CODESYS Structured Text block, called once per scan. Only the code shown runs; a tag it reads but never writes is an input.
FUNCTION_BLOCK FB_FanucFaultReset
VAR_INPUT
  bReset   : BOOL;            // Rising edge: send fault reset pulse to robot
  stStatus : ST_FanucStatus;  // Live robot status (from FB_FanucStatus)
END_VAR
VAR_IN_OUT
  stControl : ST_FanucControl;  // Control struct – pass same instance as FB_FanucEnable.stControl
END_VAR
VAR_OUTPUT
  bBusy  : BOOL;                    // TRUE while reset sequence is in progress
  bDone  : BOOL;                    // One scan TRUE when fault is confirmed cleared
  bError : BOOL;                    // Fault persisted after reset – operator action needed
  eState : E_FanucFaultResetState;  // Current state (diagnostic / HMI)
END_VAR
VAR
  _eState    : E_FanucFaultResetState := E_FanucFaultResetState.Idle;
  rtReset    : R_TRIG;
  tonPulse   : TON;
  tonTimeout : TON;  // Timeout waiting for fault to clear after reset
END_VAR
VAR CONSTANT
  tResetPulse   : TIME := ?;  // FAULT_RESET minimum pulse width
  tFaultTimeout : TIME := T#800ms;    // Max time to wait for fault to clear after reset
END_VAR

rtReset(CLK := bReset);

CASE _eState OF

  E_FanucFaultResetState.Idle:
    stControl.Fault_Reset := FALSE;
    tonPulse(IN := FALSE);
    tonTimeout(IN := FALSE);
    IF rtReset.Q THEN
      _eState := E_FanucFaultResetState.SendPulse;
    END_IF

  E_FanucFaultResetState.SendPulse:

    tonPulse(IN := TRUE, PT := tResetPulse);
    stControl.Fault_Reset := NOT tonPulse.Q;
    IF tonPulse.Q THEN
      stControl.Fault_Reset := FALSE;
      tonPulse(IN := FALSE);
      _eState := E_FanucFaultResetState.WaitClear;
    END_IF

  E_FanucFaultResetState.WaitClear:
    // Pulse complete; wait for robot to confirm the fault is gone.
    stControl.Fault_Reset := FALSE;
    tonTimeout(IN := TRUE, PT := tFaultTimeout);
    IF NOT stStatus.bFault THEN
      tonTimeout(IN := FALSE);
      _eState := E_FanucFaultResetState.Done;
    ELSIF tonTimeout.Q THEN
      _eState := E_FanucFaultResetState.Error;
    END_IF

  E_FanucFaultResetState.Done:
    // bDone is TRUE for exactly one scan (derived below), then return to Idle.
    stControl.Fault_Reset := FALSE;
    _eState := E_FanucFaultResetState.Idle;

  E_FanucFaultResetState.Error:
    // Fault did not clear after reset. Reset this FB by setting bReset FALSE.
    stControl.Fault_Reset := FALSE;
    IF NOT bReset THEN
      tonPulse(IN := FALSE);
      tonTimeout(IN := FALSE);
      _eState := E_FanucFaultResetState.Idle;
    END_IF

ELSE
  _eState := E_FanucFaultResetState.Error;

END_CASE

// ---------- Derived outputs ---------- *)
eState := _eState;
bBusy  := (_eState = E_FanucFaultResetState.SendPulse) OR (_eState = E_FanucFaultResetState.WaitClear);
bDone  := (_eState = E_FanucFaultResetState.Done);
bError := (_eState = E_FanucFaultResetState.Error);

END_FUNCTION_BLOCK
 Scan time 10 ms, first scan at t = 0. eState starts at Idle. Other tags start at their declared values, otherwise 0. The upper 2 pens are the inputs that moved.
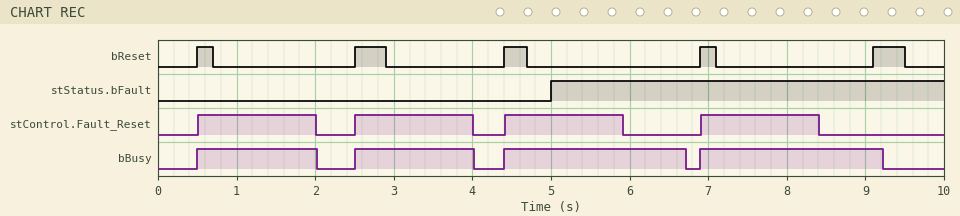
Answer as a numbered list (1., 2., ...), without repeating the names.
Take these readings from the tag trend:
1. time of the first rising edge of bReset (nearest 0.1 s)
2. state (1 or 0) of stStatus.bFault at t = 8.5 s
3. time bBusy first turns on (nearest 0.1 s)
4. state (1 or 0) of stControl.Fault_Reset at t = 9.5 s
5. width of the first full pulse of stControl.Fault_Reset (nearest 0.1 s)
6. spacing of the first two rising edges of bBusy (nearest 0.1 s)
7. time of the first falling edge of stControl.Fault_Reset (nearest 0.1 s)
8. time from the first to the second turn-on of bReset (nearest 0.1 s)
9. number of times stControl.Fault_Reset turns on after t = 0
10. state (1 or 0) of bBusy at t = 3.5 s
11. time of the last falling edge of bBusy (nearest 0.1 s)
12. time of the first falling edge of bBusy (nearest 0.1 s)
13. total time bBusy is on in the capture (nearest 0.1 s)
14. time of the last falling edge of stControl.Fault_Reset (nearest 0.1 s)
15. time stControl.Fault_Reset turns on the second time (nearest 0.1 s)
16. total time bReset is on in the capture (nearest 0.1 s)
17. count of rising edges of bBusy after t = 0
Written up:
1. 0.5 s
2. 1
3. 0.5 s
4. 0
5. 1.5 s
6. 2.0 s
7. 2.0 s
8. 2.0 s
9. 4
10. 1
11. 9.2 s
12. 2.0 s
13. 7.7 s
14. 8.4 s
15. 2.5 s
16. 1.5 s
17. 4
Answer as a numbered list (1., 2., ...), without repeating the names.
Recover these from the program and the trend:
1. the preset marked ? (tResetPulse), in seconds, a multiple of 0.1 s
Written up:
1. 1.5 s
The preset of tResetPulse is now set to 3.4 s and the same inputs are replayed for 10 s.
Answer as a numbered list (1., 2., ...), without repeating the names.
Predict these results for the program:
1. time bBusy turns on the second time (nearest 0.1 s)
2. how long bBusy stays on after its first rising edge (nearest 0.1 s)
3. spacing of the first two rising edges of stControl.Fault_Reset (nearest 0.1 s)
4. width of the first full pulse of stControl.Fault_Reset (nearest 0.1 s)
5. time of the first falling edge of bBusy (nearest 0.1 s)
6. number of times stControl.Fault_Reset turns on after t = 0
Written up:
1. 4.4 s
2. 3.4 s
3. 3.9 s
4. 3.4 s
5. 3.9 s
6. 3
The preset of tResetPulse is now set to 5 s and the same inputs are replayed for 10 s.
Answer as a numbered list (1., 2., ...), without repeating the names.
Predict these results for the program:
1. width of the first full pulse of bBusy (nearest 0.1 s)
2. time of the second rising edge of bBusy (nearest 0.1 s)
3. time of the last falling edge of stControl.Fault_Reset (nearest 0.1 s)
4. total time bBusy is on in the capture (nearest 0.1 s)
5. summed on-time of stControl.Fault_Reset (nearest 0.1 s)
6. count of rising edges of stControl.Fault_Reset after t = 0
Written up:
1. 5.8 s
2. 6.9 s
3. 5.5 s
4. 8.9 s
5. 8.1 s
6. 2
